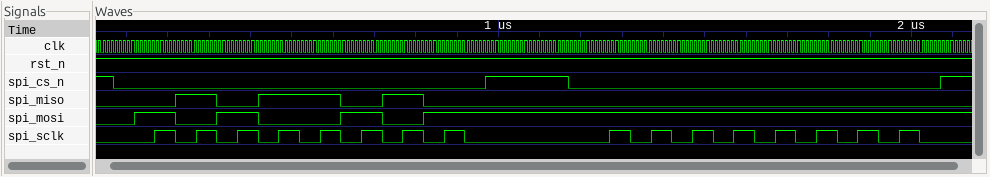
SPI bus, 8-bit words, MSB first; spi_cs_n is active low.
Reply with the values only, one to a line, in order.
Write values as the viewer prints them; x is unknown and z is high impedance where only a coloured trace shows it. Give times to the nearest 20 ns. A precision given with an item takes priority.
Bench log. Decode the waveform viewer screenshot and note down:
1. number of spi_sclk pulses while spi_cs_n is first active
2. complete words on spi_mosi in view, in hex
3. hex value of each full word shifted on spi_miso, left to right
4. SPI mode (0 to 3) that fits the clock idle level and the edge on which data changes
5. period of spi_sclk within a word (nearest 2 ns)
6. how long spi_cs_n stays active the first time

8
A5, FF
5A, 00
0
100 ns
900 ns
